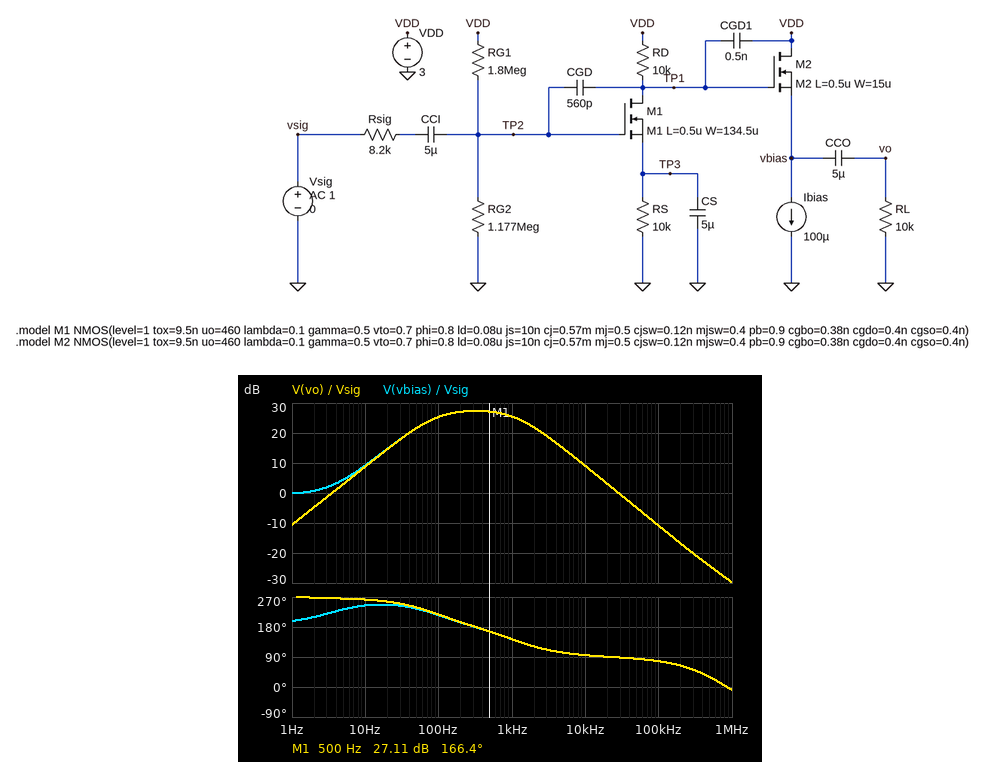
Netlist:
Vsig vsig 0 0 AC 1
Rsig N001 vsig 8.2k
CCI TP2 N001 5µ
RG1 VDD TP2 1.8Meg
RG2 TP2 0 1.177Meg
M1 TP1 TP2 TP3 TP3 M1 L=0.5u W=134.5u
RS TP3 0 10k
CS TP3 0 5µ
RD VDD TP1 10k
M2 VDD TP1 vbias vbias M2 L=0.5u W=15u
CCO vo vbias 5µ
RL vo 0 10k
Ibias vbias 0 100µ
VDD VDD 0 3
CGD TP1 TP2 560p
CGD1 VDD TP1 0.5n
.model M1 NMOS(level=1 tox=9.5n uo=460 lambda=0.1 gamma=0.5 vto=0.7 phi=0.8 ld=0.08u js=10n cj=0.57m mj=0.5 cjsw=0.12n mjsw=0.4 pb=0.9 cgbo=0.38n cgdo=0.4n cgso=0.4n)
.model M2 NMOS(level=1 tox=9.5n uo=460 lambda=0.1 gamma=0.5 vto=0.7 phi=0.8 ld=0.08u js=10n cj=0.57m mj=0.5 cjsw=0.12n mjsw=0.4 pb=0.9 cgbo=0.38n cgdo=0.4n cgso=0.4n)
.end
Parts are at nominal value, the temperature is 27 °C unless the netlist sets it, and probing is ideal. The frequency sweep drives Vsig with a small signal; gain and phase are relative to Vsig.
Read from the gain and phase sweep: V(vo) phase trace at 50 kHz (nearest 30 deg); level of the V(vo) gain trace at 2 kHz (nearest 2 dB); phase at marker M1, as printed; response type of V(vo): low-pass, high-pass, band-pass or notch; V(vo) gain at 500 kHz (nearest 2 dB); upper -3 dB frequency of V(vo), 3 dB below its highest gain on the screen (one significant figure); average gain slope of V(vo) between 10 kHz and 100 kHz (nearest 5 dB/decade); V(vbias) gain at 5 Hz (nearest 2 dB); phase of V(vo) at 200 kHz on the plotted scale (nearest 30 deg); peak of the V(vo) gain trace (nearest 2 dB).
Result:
90 deg
22 dB
166.4 deg
band-pass
-24 dB
1 kHz
-20 dB/decade
4 dB
60 deg
28 dB
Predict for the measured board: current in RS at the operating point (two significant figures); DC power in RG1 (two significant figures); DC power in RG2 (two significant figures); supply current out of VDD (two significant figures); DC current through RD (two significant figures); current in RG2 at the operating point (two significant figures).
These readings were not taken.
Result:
45 µA
1.8 µW
1.2 µW
150 µA
45 µA
1.0 µA
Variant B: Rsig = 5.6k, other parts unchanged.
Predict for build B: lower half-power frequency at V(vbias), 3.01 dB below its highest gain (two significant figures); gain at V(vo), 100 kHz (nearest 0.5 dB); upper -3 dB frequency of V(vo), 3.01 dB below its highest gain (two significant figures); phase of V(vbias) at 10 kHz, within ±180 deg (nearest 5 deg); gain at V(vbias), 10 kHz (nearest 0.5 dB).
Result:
81 Hz
-8.0 dB
1.8 kHz
100 deg
12.0 dB
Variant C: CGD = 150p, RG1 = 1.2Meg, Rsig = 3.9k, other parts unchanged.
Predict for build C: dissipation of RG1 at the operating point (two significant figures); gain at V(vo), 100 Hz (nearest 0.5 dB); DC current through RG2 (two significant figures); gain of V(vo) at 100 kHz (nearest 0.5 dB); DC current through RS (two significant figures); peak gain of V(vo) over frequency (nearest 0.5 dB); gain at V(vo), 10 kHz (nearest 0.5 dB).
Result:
1.9 µW
26.0 dB
1.3 µA
5.5 dB
74 µA
29.0 dB
24.0 dB
